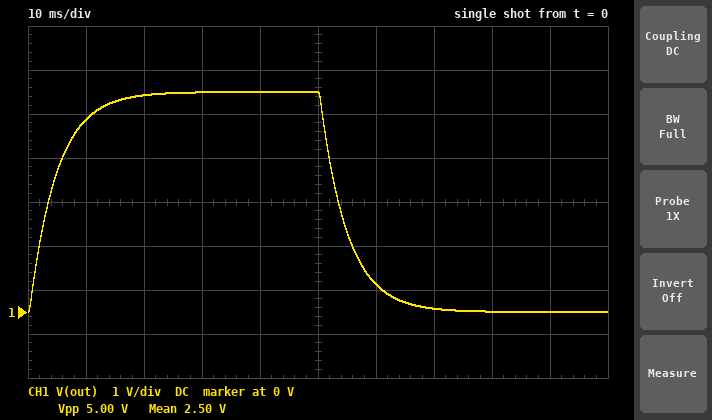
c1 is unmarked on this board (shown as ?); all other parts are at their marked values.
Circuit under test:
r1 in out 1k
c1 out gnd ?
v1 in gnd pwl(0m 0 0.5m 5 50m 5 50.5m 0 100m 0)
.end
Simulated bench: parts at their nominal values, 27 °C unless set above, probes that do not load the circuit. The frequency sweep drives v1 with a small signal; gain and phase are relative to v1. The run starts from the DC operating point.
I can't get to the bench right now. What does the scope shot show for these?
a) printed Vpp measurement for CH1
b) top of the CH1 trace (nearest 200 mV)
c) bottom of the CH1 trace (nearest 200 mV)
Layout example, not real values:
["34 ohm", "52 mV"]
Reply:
["5.00 V", "5.0 V", "0 V"]
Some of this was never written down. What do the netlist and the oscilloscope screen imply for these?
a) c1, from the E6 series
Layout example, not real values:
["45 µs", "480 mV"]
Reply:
["4.7 µF"]
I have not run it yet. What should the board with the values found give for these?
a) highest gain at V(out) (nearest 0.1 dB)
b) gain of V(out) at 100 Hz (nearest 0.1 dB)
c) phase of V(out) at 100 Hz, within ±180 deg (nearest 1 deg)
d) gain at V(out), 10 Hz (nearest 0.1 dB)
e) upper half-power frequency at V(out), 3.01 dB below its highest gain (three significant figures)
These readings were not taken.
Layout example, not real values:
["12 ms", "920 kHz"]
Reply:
["0 dB", "-9.9 dB", "-71 deg", "-0.4 dB", "33.9 Hz"]
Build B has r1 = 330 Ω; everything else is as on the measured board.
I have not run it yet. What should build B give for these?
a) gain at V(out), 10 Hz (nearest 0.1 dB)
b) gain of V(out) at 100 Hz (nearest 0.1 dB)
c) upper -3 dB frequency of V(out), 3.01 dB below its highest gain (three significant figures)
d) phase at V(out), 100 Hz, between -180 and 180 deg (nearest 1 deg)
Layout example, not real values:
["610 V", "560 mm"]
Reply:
["0 dB", "-2.9 dB", "103 Hz", "-44 deg"]
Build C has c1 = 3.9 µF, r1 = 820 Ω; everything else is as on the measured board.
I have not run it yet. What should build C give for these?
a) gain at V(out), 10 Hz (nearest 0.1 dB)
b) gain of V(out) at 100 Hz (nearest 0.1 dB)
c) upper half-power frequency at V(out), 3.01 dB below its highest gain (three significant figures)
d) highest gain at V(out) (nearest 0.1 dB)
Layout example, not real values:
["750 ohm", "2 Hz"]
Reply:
["-0.2 dB", "-7.0 dB", "49.8 Hz", "0 dB"]
